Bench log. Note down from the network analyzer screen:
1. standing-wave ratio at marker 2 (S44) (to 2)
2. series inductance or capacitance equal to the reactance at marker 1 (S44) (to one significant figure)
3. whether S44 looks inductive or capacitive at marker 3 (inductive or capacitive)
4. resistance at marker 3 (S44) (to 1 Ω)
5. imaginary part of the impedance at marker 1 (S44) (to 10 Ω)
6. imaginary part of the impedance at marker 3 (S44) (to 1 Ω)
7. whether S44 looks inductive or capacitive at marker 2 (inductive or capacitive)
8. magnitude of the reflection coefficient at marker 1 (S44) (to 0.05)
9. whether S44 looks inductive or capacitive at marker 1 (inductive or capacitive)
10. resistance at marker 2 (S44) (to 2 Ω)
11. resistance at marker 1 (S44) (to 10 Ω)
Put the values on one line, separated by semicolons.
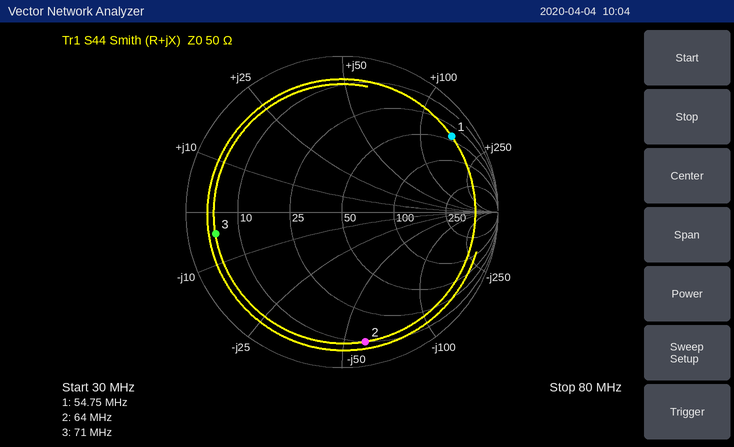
12; 400 nH; capacitive; 5 Ω; +150 Ω; -4 Ω; capacitive; 0.85; inductive; 10 Ω; 40 Ω
